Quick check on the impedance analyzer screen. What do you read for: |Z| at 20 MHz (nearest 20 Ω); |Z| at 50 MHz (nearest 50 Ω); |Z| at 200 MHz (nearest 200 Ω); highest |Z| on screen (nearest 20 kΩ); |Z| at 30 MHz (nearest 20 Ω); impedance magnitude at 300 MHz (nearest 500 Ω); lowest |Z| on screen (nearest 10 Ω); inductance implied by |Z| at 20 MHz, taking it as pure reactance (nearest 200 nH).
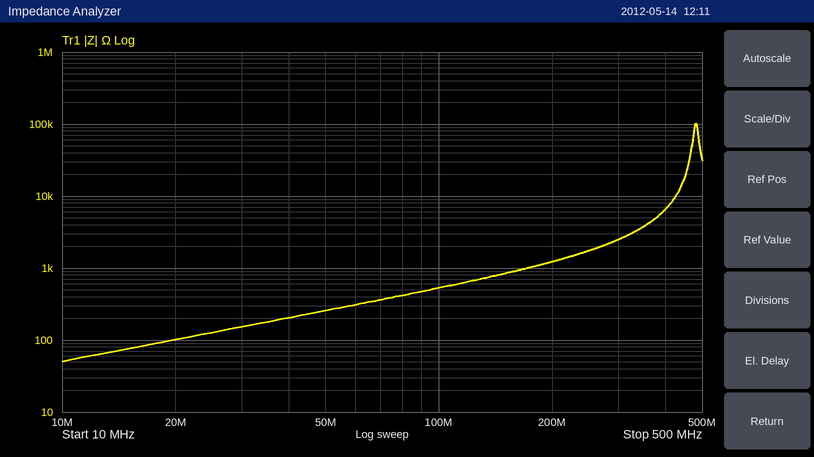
100 Ω
250 Ω
1.2 kΩ
100 kΩ
160 Ω
2.5 kΩ
50 Ω
800 nH
